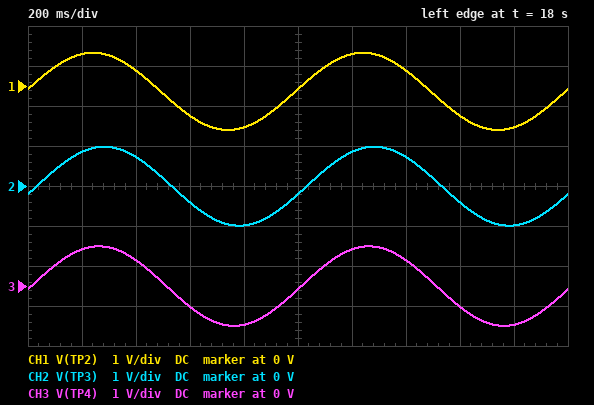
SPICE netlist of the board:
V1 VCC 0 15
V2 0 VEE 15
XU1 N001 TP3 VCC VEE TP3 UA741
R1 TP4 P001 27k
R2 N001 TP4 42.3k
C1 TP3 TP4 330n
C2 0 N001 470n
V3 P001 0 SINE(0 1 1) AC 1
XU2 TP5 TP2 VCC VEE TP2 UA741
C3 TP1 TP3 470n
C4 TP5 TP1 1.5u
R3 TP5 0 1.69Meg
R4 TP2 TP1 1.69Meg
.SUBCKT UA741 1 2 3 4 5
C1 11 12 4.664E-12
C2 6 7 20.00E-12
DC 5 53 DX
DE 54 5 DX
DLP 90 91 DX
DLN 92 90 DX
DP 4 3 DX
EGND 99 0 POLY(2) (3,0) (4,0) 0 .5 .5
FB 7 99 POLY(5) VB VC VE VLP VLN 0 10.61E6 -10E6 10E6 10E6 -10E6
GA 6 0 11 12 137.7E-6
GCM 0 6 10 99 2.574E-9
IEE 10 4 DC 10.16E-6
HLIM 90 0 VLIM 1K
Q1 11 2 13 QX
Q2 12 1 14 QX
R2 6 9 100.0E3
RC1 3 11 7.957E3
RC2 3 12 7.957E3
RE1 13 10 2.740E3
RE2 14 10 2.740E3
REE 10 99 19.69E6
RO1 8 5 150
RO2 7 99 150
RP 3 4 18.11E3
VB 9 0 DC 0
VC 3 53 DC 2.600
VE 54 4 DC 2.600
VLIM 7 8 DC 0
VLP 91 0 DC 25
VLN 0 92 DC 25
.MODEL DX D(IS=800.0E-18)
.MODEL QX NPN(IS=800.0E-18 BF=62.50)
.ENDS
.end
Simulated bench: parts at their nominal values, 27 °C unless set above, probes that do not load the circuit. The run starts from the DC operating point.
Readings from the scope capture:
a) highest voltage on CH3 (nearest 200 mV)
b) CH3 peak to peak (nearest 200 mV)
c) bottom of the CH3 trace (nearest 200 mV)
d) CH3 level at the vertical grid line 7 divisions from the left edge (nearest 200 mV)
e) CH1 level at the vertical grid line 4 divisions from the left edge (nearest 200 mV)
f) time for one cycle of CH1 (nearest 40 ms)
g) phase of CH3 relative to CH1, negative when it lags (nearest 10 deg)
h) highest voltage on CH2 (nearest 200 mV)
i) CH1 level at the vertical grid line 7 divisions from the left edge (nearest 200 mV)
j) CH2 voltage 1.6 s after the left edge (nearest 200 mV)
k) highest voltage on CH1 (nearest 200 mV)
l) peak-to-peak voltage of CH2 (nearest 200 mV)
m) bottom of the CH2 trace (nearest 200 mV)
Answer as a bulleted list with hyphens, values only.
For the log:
- 1.0 V
- 2.0 V
- -1.0 V
- 600 mV
- -1.0 V
- 1.00 s
- -10 deg
- 1.0 V
- 400 mV
- -400 mV
- 800 mV
- 2.0 V
- -1.0 V
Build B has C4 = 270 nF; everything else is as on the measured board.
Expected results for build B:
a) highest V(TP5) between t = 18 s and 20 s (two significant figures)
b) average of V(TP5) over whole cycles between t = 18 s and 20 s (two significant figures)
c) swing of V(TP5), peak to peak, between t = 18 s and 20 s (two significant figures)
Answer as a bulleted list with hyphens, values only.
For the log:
- 780 mV
- -130 mV
- 1.8 V
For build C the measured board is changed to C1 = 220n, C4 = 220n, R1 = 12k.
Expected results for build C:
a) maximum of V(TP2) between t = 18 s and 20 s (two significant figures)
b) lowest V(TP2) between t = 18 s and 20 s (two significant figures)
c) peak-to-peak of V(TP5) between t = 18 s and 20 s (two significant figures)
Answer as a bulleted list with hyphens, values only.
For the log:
- 760 mV
- -1.0 V
- 1.8 V
